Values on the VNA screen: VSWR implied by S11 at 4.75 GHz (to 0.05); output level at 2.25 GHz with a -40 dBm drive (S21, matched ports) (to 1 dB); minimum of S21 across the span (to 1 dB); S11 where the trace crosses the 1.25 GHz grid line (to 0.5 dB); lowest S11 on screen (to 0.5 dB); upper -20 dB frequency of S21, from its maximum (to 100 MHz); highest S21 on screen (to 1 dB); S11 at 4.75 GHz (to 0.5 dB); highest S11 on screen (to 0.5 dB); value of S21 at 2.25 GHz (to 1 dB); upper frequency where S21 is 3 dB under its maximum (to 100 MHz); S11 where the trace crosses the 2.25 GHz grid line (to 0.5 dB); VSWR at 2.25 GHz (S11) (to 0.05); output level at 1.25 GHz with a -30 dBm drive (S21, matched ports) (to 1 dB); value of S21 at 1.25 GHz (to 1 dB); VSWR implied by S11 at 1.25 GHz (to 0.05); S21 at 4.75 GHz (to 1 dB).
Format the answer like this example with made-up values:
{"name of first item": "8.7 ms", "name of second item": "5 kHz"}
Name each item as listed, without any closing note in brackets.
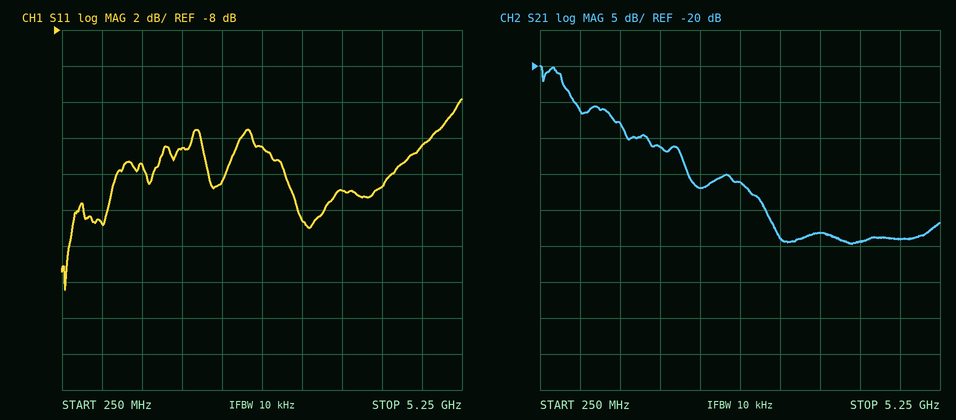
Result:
{"VSWR implied by S11 at 4.75 GHz": "1.45", "output level at 2.25 GHz with a -40 dBm drive (S21, matched ports)": "-77 dBm", "minimum of S21 across the span": "-45 dB", "S11 where the trace crosses the 1.25 GHz grid line": "-15.5 dB", "lowest S11 on screen": "-22.5 dB", "upper -20 dB frequency of S21, from its maximum": "3.1 GHz", "highest S21 on screen": "-20 dB", "S11 at 4.75 GHz": "-14.5 dB", "highest S11 on screen": "-12.0 dB", "value of S21 at 2.25 GHz": "-37 dB", "upper frequency where S21 is 3 dB under its maximum": "600 MHz", "S11 where the trace crosses the 2.25 GHz grid line": "-16.5 dB", "VSWR at 2.25 GHz (S11)": "1.35", "output level at 1.25 GHz with a -30 dBm drive (S21, matched ports)": "-58 dBm", "value of S21 at 1.25 GHz": "-28 dB", "VSWR implied by S11 at 1.25 GHz": "1.40", "S21 at 4.75 GHz": "-44 dB"}
